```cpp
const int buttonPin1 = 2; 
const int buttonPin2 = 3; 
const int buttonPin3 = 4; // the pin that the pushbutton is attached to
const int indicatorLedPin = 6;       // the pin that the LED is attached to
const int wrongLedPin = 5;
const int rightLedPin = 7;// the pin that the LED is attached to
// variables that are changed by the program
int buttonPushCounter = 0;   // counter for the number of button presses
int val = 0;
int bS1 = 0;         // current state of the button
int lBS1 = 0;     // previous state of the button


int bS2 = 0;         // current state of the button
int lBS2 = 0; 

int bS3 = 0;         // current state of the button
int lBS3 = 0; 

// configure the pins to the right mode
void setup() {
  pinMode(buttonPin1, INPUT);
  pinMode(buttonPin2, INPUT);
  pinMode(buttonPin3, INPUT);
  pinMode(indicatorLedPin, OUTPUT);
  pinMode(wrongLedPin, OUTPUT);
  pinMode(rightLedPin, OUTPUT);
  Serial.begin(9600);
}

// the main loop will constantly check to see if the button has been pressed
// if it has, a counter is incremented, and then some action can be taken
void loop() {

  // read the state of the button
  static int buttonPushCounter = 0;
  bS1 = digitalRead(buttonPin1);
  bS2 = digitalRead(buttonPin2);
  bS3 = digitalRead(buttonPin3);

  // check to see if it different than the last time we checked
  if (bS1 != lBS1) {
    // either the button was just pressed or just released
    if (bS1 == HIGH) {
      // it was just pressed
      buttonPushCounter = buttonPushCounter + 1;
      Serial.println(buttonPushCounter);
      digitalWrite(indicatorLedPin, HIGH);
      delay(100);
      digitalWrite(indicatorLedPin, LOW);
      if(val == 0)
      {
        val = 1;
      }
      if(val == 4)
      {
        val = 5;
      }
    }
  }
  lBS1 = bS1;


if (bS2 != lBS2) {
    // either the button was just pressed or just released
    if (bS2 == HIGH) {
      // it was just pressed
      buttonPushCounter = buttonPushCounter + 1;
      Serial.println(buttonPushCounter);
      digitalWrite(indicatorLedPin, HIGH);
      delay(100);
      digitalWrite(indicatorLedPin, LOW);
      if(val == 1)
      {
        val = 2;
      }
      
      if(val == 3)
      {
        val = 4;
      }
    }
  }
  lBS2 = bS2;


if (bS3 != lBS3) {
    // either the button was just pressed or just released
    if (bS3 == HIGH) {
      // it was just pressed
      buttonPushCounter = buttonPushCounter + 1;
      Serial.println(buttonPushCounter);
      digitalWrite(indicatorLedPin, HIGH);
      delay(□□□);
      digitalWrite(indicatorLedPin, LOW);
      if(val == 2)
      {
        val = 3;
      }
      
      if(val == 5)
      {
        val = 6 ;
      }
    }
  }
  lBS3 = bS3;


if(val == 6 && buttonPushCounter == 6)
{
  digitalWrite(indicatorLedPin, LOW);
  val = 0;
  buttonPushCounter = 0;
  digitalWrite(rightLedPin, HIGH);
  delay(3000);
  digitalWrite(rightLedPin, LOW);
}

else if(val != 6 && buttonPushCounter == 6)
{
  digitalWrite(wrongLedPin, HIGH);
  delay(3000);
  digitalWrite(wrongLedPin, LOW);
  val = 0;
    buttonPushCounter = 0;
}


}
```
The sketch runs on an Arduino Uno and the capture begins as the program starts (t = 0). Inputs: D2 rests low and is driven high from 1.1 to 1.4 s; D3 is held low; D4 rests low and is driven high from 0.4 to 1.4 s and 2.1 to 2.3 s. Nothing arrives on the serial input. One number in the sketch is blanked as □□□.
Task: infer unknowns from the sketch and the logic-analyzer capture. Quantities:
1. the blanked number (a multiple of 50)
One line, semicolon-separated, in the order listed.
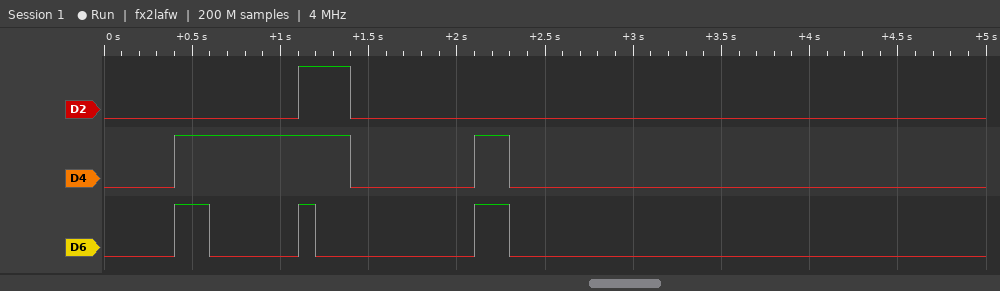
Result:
200
